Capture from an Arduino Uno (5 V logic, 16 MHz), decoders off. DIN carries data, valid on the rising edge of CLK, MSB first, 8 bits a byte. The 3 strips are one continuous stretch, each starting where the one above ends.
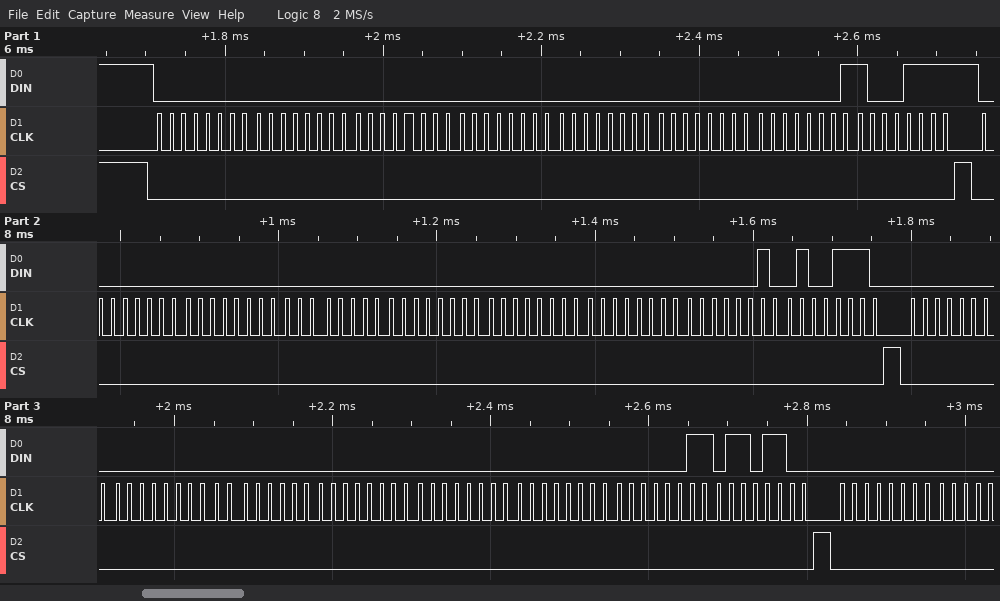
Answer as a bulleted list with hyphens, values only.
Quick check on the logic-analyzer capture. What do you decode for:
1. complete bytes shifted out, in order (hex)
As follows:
- 00 00 00 00 00 00 01 8F 00 00 00 00 00 00 02 4E 00 00 00 00 00 00 03 6C 00
